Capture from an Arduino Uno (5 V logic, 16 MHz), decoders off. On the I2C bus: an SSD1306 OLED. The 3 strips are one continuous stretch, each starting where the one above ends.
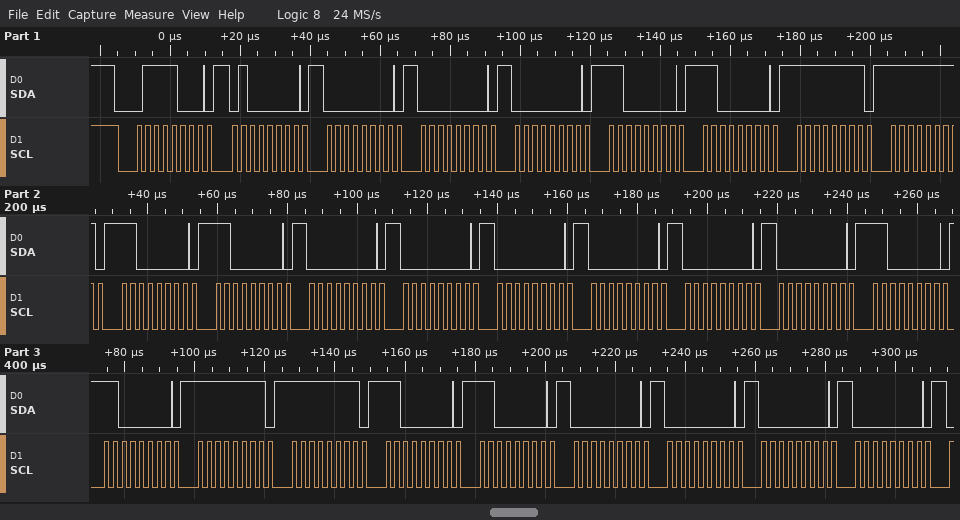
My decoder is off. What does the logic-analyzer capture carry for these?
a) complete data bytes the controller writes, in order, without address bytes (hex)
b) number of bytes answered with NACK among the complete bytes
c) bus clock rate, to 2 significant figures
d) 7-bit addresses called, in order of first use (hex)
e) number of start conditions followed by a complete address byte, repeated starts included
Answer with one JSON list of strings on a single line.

["40 00 00 00 C0 C0 FF FF C0 C0 00 00 00 00 00 00 C0 C0 FF FF C0 C0 00 00 00 00", "0", "400 kHz", "0x3C", "1"]
